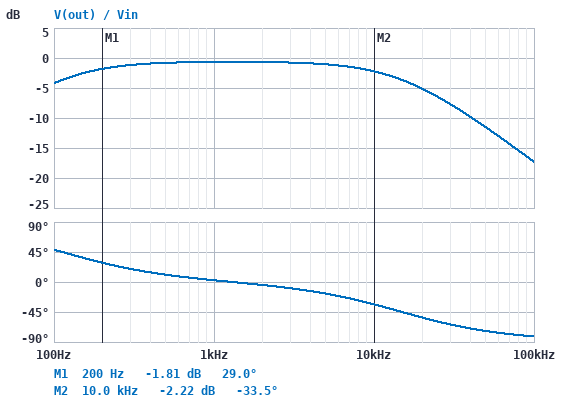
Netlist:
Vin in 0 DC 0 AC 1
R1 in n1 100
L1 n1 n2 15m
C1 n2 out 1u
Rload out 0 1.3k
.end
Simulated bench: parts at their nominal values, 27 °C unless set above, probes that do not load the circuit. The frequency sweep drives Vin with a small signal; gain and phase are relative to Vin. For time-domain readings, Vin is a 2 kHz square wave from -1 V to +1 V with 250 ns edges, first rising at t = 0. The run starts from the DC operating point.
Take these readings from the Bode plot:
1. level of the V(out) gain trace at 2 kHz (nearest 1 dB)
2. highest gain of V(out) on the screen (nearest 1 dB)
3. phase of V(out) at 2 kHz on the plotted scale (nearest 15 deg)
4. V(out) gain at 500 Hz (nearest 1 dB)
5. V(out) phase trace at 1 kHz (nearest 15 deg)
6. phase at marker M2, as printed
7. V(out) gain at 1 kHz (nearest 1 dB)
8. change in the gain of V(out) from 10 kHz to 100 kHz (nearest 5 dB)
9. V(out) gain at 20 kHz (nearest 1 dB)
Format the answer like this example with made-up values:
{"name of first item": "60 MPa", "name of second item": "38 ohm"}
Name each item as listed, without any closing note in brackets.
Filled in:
{"level of the V(out) gain trace at 2 kHz": "-1 dB", "highest gain of V(out) on the screen": "-1 dB", "phase of V(out) at 2 kHz on the plotted scale": "0 deg", "V(out) gain at 500 Hz": "-1 dB", "V(out) phase trace at 1 kHz": "0 deg", "phase at marker M2, as printed": "-33.5 deg", "V(out) gain at 1 kHz": "-1 dB", "change in the gain of V(out) from 10 kHz to 100 kHz": "-15 dB", "V(out) gain at 20 kHz": "-5 dB"}
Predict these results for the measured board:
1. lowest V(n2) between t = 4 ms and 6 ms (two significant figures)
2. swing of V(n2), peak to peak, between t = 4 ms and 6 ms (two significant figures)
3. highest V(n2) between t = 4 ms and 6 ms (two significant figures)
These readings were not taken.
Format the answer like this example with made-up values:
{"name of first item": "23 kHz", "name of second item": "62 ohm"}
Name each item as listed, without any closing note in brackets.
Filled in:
{"lowest V(n2) between t = 4 ms and 6 ms": "-940 mV", "swing of V(n2), peak to peak, between t = 4 ms and 6 ms": "1.9 V", "highest V(n2) between t = 4 ms and 6 ms": "940 mV"}
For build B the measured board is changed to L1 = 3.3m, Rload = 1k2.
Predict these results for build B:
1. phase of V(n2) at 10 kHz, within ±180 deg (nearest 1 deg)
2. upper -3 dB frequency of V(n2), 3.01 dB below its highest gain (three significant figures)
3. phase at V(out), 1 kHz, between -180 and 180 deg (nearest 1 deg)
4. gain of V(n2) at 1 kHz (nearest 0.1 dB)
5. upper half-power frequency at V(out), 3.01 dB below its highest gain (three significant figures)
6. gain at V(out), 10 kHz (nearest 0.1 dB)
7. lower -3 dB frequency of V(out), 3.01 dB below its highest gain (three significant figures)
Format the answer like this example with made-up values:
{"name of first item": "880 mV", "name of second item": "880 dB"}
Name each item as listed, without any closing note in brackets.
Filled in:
{"phase of V(n2) at 10 kHz, within ±180 deg": "-9 deg", "upper -3 dB frequency of V(n2), 3.01 dB below its highest gain": "52.8 kHz", "phase at V(out), 1 kHz, between -180 and 180 deg": "6 deg", "gain of V(n2) at 1 kHz": "-0.7 dB", "upper half-power frequency at V(out), 3.01 dB below its highest gain": "62.8 kHz", "gain at V(out), 10 kHz": "-0.8 dB", "lower -3 dB frequency of V(out), 3.01 dB below its highest gain": "122 Hz"}
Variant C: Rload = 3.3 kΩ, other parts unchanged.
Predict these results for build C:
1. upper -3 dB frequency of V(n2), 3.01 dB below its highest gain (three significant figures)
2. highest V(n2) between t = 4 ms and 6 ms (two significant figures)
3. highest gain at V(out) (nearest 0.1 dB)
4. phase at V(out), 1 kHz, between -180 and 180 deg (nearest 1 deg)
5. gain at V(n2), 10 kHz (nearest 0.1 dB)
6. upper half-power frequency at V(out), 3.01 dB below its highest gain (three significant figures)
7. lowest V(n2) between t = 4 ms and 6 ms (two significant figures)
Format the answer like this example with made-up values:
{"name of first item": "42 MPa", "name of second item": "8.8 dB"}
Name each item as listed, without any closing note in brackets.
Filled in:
{"upper -3 dB frequency of V(n2), 3.01 dB below its highest gain": "34.0 kHz", "highest V(n2) between t = 4 ms and 6 ms": "970 mV", "highest gain at V(out)": "-0.3 dB", "phase at V(out), 1 kHz, between -180 and 180 deg": "1 deg", "gain at V(n2), 10 kHz": "-0.6 dB", "upper half-power frequency at V(out), 3.01 dB below its highest gain": "36.1 kHz", "lowest V(n2) between t = 4 ms and 6 ms": "-980 mV"}
